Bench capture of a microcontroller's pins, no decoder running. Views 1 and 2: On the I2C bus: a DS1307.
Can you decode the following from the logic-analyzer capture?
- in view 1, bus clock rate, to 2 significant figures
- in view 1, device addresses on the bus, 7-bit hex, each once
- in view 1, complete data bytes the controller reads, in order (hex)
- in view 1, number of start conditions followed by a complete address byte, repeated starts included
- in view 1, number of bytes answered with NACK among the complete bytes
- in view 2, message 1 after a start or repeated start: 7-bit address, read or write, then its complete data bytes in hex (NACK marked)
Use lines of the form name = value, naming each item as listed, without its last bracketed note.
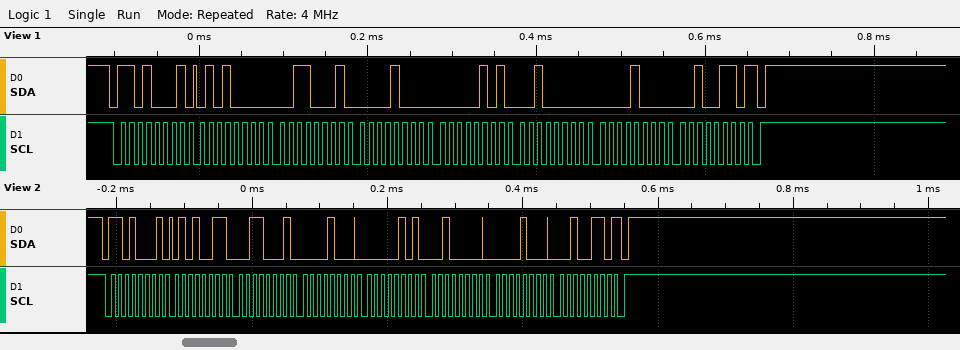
in view 1, bus clock rate, to 2 significant figures = 100 kHz
in view 1, device addresses on the bus, 7-bit hex, each once = 0x68
in view 1, complete data bytes the controller reads, in order = 50 31 08 05 20 08 26
in view 1, number of start conditions followed by a complete address byte, repeated starts included = 1
in view 1, number of bytes answered with NACK among the complete bytes = 1
in view 2, message 1 after a start or repeated start: 7-bit address, read or write, then its complete data bytes in hex = 0x68 read: 53 31 08 05 20 08 26 NACK
